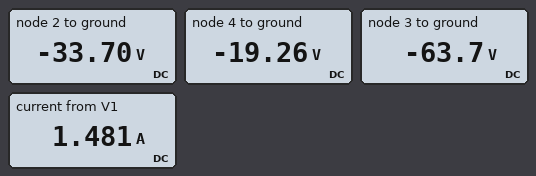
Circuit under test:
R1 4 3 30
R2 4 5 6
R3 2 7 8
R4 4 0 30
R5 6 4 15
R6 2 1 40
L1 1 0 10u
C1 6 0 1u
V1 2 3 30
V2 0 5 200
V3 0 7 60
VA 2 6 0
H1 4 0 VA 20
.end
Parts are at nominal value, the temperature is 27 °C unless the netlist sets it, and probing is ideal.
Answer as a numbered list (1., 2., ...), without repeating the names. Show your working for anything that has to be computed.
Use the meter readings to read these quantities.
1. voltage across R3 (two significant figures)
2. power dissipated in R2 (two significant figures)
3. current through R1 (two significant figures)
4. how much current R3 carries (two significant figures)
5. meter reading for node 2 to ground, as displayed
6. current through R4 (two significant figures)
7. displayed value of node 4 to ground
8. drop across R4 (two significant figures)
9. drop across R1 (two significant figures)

1. -33.7 V - (-60 V) = 26 V
2. (-19.26 V - (-200 V))^2 / 6 Ω = 5.4 kW
3. (-19.26 V - (-63.7 V)) / 30 Ω = 1.5 A
4. (-33.7 V - (-60 V)) / 8 Ω = 3.3 A
5. -33.70 V
6. (0 V - (-19.26 V)) / 30 Ω = 640 mA
7. -19.26 V
8. 0 V - (-19.26 V) = 19 V
9. -19.26 V - (-63.7 V) = 44 V
